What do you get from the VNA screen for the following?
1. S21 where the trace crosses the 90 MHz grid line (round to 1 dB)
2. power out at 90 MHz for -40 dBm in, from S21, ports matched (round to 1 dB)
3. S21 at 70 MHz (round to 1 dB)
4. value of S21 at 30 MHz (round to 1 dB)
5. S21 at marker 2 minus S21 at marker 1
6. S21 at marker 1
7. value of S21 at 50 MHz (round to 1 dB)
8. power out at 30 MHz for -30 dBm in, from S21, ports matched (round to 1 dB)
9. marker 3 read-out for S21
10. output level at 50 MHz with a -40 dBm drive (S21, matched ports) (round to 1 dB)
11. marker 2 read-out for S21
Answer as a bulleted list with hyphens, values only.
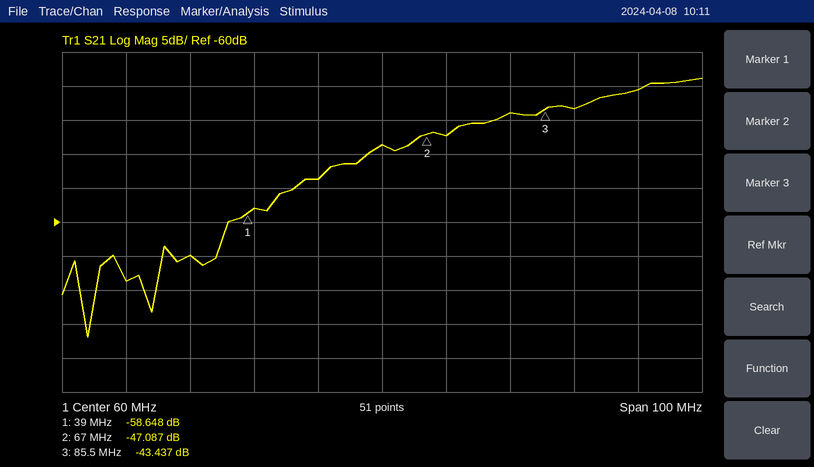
- -43 dB
- -83 dBm
- -47 dB
- -65 dB
- 11.561 dB
- -58.648 dB
- -54 dB
- -95 dBm
- -43.437 dB
- -94 dBm
- -47.087 dB
